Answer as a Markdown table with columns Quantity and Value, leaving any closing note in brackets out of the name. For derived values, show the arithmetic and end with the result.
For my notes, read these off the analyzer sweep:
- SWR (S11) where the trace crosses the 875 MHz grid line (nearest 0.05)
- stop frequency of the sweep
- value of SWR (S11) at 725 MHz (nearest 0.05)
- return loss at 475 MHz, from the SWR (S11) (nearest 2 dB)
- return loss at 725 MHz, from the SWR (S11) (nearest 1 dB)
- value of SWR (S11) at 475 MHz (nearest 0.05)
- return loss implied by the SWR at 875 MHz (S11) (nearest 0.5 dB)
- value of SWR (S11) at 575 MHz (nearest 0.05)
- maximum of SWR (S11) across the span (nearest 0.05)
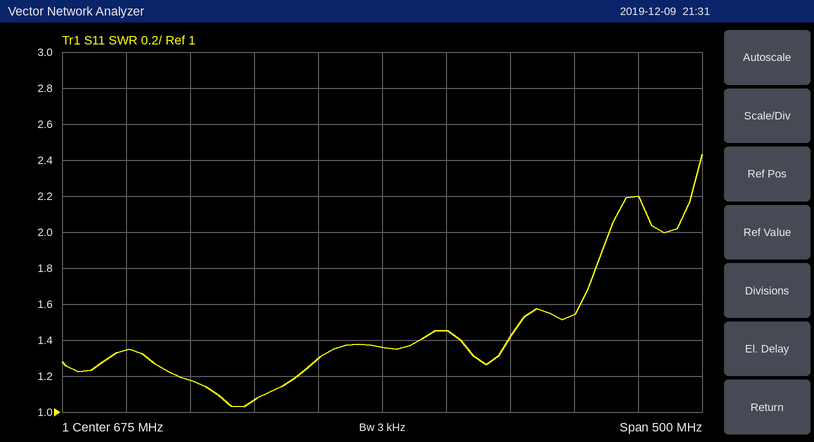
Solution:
| Quantity | Value |
|---|---|
| SWR (S11) where the trace crosses the 875 MHz grid line | 2.20 |
| stop frequency of the sweep | 925 MHz |
| value of SWR (S11) at 725 MHz | 1.45 |
| return loss at 475 MHz, from the SWR (S11) | −20 log10((1.35 − 1)/(1.35 + 1)) ≈ 16 dB |
| return loss at 725 MHz, from the SWR (S11) | −20 log10((1.45 − 1)/(1.45 + 1)) ≈ 15 dB |
| value of SWR (S11) at 475 MHz | 1.35 |
| return loss implied by the SWR at 875 MHz (S11) | −20 log10((2.2 − 1)/(2.2 + 1)) ≈ 8.5 dB |
| value of SWR (S11) at 575 MHz | 1.05 |
| maximum of SWR (S11) across the span | 2.45 |
